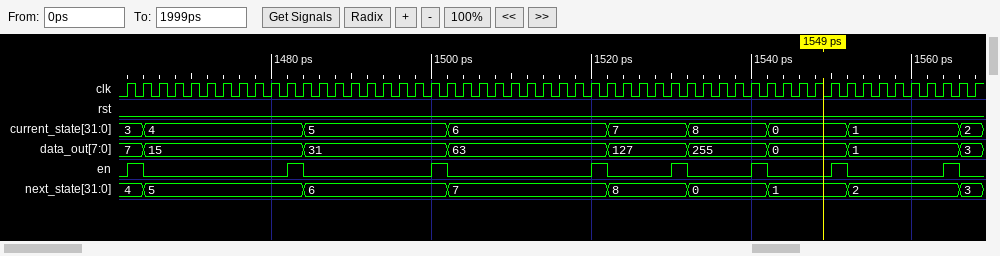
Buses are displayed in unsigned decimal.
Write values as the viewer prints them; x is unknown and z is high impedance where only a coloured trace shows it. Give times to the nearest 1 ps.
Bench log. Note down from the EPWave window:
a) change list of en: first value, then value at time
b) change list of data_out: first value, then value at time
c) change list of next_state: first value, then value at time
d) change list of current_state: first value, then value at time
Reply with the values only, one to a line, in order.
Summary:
0, 1 at 1462 ps, 0 at 1464 ps, 1 at 1482 ps, 0 at 1484 ps, 1 at 1500 ps, 0 at 1502 ps, 1 at 1520 ps, 0 at 1522 ps, 1 at 1530 ps, 0 at 1532 ps, 1 at 1540 ps, 0 at 1542 ps, 1 at 1550 ps, 0 at 1552 ps, 1 at 1564 ps, 0 at 1566 ps
7, 15 at 1464 ps, 31 at 1484 ps, 63 at 1502 ps, 127 at 1522 ps, 255 at 1532 ps, 0 at 1542 ps, 1 at 1552 ps, 3 at 1566 ps
4, 5 at 1464 ps, 6 at 1484 ps, 7 at 1502 ps, 8 at 1522 ps, 0 at 1532 ps, 1 at 1542 ps, 2 at 1552 ps, 3 at 1566 ps
3, 4 at 1464 ps, 5 at 1484 ps, 6 at 1502 ps, 7 at 1522 ps, 8 at 1532 ps, 0 at 1542 ps, 1 at 1552 ps, 2 at 1566 ps
